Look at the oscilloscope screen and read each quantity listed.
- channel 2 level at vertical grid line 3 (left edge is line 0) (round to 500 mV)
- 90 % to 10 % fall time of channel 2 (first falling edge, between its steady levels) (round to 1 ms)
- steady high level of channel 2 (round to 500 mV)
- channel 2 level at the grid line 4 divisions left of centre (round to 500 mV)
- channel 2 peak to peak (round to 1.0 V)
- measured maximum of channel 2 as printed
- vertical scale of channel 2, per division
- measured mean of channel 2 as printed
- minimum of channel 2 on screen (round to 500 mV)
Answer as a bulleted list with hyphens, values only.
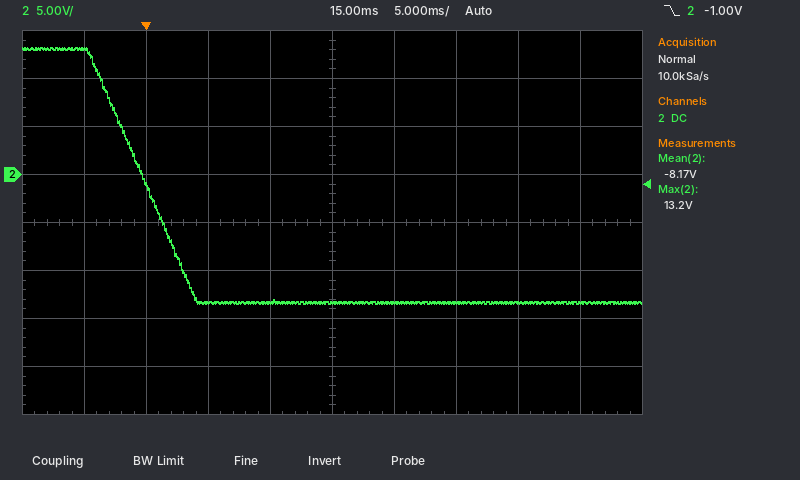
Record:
- -13.5 V
- 7 ms
- 13.0 V
- 13.0 V
- 27.0 V
- 13.2 V
- 5 V
- -8.17 V
- -13.5 V
